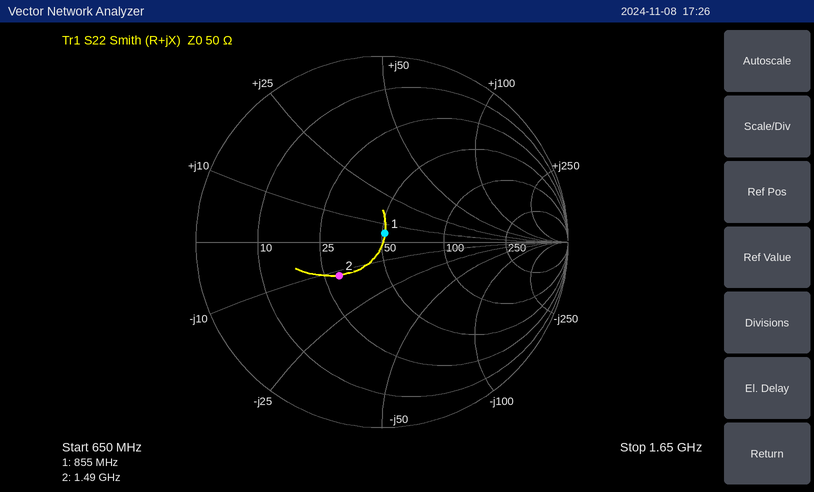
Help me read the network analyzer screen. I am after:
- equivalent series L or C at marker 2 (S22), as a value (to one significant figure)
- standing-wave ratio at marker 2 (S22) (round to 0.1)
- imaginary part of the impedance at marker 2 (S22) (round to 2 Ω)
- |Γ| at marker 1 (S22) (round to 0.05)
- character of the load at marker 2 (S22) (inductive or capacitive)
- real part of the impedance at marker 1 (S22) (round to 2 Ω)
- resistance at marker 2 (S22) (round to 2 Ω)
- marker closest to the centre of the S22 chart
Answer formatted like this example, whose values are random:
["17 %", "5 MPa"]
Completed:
["9 pF", "1.8", "-12 Ω", "0.05", "capacitive", "52 Ω", "30 Ω", "marker 1"]
